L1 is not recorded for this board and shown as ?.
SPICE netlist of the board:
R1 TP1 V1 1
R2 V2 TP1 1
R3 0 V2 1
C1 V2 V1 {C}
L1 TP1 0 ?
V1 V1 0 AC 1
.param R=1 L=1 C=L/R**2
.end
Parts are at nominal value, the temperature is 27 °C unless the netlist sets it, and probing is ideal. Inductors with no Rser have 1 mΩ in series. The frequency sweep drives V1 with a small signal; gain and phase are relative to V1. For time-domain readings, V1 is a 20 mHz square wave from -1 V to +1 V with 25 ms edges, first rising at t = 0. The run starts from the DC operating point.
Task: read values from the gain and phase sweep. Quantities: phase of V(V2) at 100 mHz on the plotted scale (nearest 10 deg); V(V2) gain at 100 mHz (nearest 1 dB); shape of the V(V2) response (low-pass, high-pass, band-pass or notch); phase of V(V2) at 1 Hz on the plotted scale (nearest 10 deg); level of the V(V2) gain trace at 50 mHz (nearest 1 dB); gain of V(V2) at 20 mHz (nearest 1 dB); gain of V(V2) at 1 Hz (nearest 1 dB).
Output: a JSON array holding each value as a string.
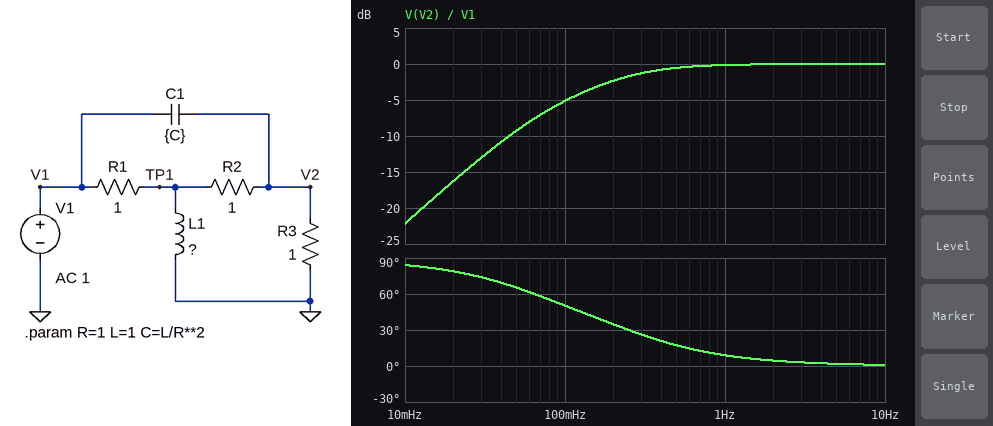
["50 deg", "-5 dB", "high-pass", "10 deg", "-9 dB", "-16 dB", "0 dB"]
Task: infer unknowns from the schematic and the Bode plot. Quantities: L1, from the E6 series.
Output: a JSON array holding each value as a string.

["1.5 H"]
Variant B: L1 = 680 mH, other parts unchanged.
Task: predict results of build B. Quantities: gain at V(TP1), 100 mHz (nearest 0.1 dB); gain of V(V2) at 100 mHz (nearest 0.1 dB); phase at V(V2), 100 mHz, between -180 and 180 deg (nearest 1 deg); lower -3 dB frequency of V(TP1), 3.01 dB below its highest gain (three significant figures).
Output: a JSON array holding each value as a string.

["-7.6 dB", "-6.2 dB", "64 deg", "195 mHz"]
